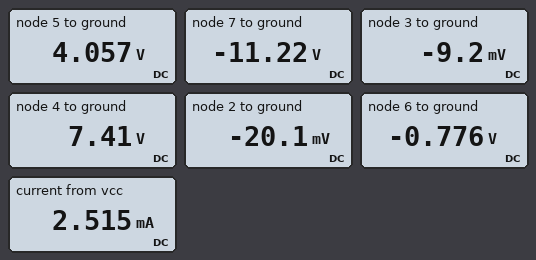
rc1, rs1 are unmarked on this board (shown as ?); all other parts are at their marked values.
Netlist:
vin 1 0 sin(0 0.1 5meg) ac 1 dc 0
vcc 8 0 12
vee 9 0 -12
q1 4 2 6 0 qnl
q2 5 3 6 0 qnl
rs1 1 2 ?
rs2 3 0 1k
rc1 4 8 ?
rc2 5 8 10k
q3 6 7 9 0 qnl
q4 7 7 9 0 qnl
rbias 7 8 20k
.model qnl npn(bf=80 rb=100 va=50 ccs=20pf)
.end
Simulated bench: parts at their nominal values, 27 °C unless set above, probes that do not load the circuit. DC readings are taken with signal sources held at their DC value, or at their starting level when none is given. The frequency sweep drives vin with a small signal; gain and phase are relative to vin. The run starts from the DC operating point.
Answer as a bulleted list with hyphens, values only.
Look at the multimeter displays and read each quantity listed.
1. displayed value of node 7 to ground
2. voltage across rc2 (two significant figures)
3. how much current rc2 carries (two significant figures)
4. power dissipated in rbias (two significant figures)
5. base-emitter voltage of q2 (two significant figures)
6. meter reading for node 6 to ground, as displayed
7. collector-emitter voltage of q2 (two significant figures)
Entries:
- -11.22 V
- 7.9 V
- 790 µA
- 27 mW
- 770 mV
- -0.776 V
- 4.8 V
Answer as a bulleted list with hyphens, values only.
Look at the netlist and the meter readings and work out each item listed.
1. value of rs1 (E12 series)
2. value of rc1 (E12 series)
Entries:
- 3.3 kΩ
- 8.2 kΩ
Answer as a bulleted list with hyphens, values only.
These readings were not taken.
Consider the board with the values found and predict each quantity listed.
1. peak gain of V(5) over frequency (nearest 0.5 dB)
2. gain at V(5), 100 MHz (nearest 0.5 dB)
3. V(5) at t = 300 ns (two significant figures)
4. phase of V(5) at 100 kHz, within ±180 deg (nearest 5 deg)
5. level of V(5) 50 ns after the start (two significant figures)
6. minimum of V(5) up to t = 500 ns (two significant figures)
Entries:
- 37.0 dB
- -4.5 dB
- 5.6 V
- -5 deg
- 5.1 V
- 3.5 V
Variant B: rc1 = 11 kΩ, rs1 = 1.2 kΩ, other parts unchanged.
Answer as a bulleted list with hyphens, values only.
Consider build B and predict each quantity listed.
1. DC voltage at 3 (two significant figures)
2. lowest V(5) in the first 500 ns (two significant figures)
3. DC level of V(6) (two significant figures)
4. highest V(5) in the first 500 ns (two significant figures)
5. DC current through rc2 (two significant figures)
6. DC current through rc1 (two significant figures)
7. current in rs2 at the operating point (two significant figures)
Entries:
- -7.9 mV
- 4.1 V
- -770 mV
- 6.9 V
- 690 µA
- 660 µA
- 7.9 µA
